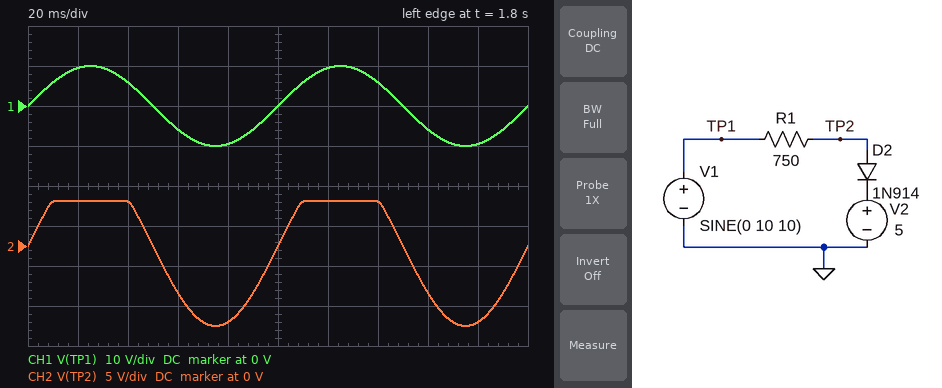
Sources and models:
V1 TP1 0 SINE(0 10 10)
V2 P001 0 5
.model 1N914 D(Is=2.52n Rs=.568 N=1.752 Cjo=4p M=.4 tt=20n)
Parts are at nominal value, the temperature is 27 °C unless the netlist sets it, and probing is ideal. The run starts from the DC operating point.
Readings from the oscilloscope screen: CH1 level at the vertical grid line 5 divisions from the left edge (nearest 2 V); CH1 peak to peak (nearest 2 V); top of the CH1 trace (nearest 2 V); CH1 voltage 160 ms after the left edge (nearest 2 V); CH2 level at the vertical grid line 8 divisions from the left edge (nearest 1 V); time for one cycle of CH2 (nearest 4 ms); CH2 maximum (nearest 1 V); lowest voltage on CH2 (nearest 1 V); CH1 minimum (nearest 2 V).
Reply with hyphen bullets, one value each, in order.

- 0 V
- 20 V
- 10 V
- -6 V
- -6 V
- 100 ms
- 6 V
- -10 V
- -10 V
